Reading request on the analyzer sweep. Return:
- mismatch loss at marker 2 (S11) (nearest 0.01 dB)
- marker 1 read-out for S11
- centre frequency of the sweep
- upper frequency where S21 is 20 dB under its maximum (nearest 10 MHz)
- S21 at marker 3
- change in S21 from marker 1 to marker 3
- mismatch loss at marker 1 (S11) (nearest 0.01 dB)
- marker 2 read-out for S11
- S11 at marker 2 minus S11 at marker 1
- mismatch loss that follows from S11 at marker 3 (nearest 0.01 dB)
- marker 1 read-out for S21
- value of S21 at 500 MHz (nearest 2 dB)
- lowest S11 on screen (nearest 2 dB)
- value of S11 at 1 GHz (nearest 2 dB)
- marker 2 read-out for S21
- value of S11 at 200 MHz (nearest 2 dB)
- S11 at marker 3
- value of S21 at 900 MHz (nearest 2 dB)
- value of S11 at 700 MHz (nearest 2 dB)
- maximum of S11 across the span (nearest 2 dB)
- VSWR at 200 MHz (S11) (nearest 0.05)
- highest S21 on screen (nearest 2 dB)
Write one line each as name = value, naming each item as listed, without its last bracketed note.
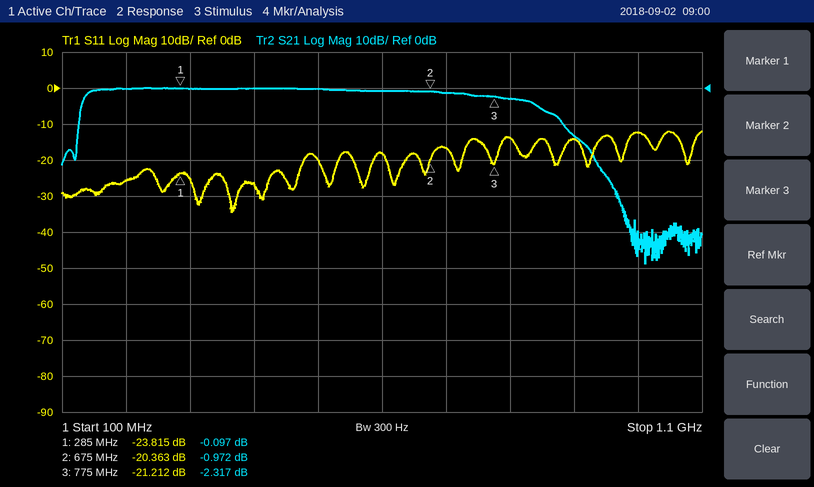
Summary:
mismatch loss at marker 2 (S11) = 0.04 dB
marker 1 read-out for S11 = -23.815 dB
centre frequency of the sweep = 600 MHz
upper frequency where S21 is 20 dB under its maximum = 930 MHz
S21 at marker 3 = -2.317 dB
change in S21 from marker 1 to marker 3 = -2.220 dB
mismatch loss at marker 1 (S11) = 0.02 dB
marker 2 read-out for S11 = -20.363 dB
S11 at marker 2 minus S11 at marker 1 = 3.452 dB
mismatch loss that follows from S11 at marker 3 = 0.03 dB
marker 1 read-out for S21 = -0.097 dB
value of S21 at 500 MHz = 0 dB
lowest S11 on screen = -34 dB
value of S11 at 1 GHz = -12 dB
marker 2 read-out for S21 = -0.972 dB
value of S11 at 200 MHz = -26 dB
S11 at marker 3 = -21.212 dB
value of S21 at 900 MHz = -14 dB
value of S11 at 700 MHz = -16 dB
maximum of S11 across the span = -12 dB
VSWR at 200 MHz (S11) = 1.10
highest S21 on screen = 0 dB
